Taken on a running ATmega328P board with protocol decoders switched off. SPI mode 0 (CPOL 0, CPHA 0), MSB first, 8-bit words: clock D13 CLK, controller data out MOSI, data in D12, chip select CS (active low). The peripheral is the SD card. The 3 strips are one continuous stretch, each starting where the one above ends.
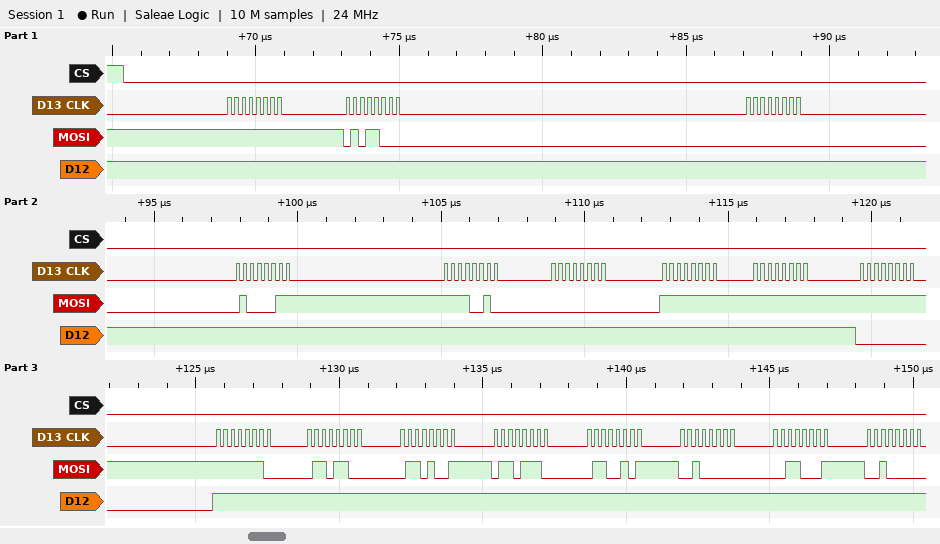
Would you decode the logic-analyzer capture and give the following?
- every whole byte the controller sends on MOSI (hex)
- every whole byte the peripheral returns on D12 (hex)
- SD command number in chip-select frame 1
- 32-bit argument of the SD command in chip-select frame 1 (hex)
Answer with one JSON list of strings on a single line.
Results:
["0xFF 0x58 0x00 0x43 0xF2 0x00 0xFF 0xFF 0xFF 0xFE 0x6C 0x69 0x6E 0x65 0x20 0x31 0x20", "0xFF 0xFF 0xFF 0xFF 0xFF 0xFF 0xFF 0xFF 0x00 0xFF 0xFF 0xFF 0xFF 0xFF 0xFF 0xFF 0xFF", "CMD24", "0x0043F200"]
